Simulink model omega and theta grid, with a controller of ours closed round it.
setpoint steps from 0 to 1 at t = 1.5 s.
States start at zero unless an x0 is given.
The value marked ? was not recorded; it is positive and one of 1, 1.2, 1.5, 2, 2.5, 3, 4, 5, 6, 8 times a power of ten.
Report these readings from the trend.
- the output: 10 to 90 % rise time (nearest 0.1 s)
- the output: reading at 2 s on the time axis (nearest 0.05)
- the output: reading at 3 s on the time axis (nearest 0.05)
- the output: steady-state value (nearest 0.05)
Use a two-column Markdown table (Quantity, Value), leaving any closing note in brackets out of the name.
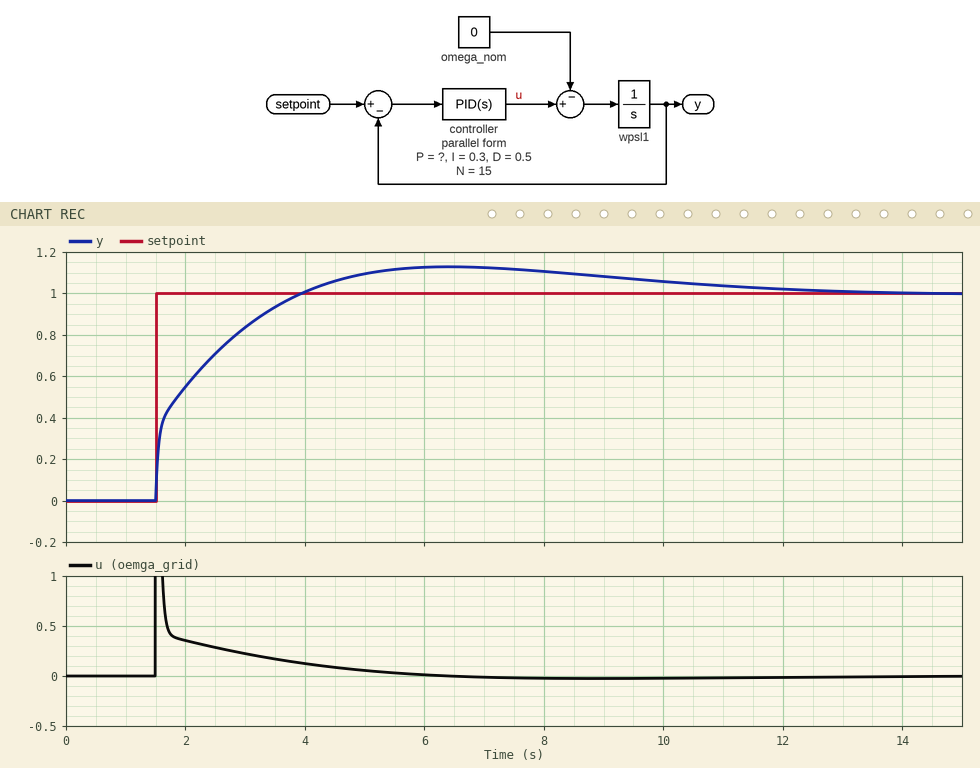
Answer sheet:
| Quantity | Value |
|---|---|
| the output: 10 to 90 % rise time | 1.8 s |
| the output: reading at 2 s on the time axis | 0.55 |
| the output: reading at 3 s on the time axis | 0.85 |
| the output: steady-state value | 1.00 |
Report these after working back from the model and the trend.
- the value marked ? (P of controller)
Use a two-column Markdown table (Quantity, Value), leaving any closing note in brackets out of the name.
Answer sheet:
| Quantity | Value |
|---|---|
| the value marked ? | 1 |
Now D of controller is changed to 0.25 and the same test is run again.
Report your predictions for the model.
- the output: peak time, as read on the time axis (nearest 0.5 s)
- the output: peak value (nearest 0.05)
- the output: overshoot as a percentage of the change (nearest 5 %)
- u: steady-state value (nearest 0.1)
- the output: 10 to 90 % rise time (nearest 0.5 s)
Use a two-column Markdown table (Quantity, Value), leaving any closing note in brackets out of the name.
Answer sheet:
| Quantity | Value |
|---|---|
| the output: peak time, as read on the time axis | 6.0 s |
| the output: peak value | 1.15 |
| the output: overshoot as a percentage of the change | 15 % |
| u: steady-state value | 0.0 |
| the output: 10 to 90 % rise time | 1.5 s |
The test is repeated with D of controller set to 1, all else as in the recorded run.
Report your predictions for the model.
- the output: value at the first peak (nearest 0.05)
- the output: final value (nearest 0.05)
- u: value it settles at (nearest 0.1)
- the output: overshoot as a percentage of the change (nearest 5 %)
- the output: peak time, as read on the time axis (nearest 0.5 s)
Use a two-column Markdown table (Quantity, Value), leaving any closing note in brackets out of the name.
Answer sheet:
| Quantity | Value |
|---|---|
| the output: value at the first peak | 1.10 |
| the output: final value | 1.00 |
| u: value it settles at | 0.0 |
| the output: overshoot as a percentage of the change | 10 % |
| the output: peak time, as read on the time axis | 7.5 s |
